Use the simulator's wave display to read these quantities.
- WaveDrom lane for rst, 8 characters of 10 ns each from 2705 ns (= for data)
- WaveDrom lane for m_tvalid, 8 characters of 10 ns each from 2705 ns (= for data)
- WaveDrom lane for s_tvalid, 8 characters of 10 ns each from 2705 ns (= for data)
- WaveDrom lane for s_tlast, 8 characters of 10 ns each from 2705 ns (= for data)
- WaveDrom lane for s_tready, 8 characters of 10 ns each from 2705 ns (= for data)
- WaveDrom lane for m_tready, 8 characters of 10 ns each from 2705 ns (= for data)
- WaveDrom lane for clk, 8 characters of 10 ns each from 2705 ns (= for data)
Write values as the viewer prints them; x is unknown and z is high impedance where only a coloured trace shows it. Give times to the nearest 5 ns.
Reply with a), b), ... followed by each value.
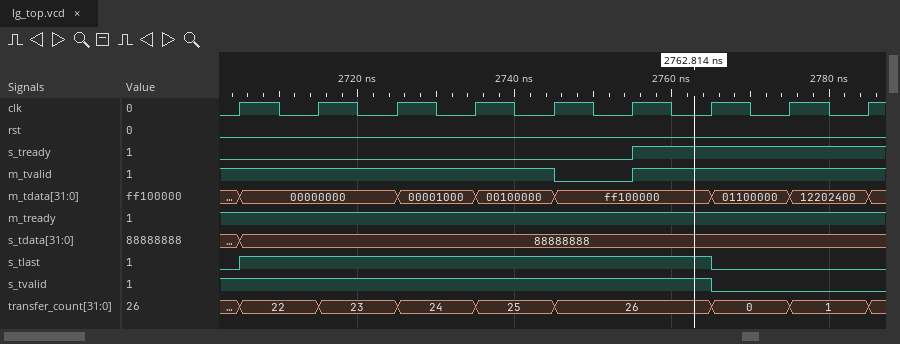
a) {name: 'rst', wave: '0.......'}
b) {name: 'm_tvalid', wave: '1...01..'}
c) {name: 's_tvalid', wave: '1.....0.'}
d) {name: 's_tlast', wave: '1.....0.'}
e) {name: 's_tready', wave: '0....1..'}
f) {name: 'm_tready', wave: '1.......'}
g) {name: 'clk', wave: 'p.......'}
